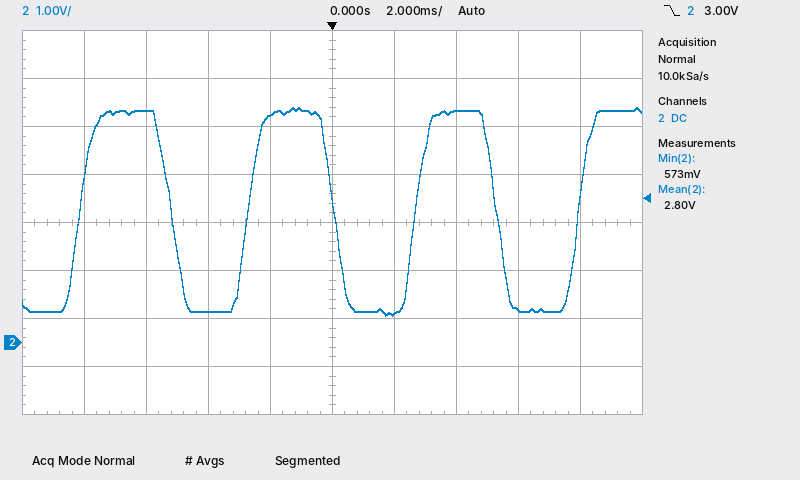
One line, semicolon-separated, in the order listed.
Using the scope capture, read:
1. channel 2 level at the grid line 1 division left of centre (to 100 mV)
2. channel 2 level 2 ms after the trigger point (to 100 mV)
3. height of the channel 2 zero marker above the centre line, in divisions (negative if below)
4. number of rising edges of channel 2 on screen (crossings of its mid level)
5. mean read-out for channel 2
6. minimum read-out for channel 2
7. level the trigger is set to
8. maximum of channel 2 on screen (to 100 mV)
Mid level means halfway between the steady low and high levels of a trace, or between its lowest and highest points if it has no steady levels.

4.7 V; 600 mV; -2.5 div; 4; 2.80 V; 573 mV; 3.00 V; 4.9 V
